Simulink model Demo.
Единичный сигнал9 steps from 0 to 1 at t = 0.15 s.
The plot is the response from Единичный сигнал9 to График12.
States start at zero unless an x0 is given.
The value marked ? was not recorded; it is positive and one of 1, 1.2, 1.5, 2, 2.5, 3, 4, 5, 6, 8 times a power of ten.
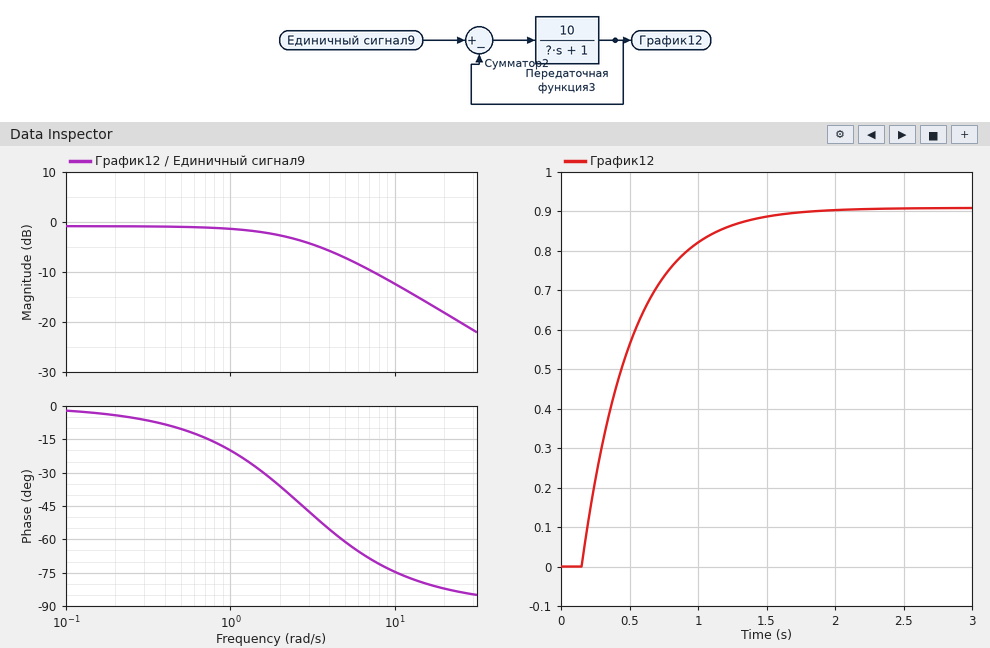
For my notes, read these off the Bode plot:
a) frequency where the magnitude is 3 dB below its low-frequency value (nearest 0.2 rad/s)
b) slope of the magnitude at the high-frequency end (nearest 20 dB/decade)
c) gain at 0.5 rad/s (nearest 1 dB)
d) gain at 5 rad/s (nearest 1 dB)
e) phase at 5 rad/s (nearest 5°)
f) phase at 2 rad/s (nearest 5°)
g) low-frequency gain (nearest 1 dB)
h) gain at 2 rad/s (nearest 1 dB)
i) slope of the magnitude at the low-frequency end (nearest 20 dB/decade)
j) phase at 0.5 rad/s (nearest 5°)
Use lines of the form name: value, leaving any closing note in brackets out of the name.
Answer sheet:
frequency where the magnitude is 3 dB below its low-frequency value: 2.8 rad/s
slope of the magnitude at the high-frequency end: -20 dB/decade
gain at 0.5 rad/s: -1 dB
gain at 5 rad/s: -7 dB
phase at 5 rad/s: -60°
phase at 2 rad/s: -35°
low-frequency gain: -1 dB
gain at 2 rad/s: -3 dB
slope of the magnitude at the low-frequency end: 0 dB/decade
phase at 0.5 rad/s: -10°
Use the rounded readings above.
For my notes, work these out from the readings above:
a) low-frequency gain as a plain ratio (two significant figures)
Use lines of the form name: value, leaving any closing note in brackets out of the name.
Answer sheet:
low-frequency gain as a plain ratio: 0.89
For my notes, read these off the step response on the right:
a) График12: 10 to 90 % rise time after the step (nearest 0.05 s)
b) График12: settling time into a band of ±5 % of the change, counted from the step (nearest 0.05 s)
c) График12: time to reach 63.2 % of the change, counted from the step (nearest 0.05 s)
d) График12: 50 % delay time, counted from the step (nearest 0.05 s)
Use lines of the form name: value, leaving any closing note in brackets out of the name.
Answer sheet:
График12: 10 to 90 % rise time after the step: 0.80 s
График12: settling time into a band of ±5 % of the change, counted from the step: 1.10 s
График12: time to reach 63.2 % of the change, counted from the step: 0.35 s
График12: 50 % delay time, counted from the step: 0.25 s
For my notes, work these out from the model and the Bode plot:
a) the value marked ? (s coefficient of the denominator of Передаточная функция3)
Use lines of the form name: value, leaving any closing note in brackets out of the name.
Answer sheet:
the value marked ?: 4
